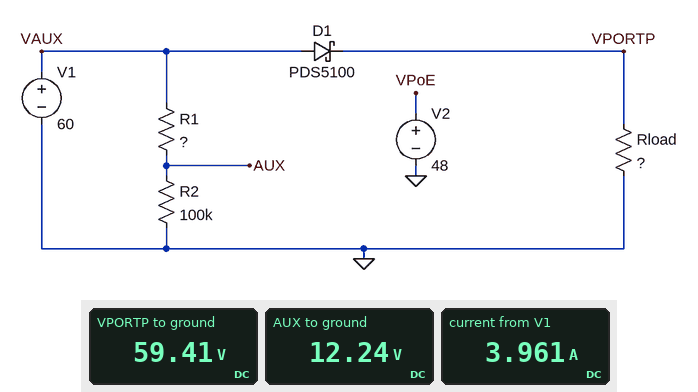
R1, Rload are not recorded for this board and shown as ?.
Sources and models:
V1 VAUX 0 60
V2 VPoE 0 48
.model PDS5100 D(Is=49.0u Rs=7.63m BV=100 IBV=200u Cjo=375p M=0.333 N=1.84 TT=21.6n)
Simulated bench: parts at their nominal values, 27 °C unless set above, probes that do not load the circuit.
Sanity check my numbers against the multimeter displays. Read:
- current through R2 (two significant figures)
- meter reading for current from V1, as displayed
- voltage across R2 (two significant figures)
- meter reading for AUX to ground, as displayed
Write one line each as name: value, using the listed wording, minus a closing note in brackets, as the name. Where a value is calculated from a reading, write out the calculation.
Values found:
current through R2: (12.24 V) / 100 kΩ = 120 µA
meter reading for current from V1, as displayed: 3.961 A
voltage across R2: 12.24 V = 12 V
meter reading for AUX to ground, as displayed: 12.24 V
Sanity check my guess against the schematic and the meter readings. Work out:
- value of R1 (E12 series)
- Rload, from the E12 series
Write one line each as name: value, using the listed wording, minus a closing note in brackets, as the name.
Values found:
value of R1: 390 kΩ
Rload, from the E12 series: 15 Ω
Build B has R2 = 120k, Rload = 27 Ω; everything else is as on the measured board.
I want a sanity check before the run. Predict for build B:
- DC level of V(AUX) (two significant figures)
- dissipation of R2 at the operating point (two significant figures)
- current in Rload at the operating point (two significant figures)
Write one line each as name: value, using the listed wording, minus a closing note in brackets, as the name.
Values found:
DC level of V(AUX): 14 V
dissipation of R2 at the operating point: 1.7 mW
current in Rload at the operating point: 2.2 A
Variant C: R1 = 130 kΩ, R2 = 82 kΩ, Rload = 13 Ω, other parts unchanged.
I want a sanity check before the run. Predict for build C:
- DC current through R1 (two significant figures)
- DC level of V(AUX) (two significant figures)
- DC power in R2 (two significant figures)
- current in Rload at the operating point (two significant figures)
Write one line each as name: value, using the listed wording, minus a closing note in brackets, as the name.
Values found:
DC current through R1: 280 µA
DC level of V(AUX): 23 V
DC power in R2: 6.6 mW
current in Rload at the operating point: 4.6 A
